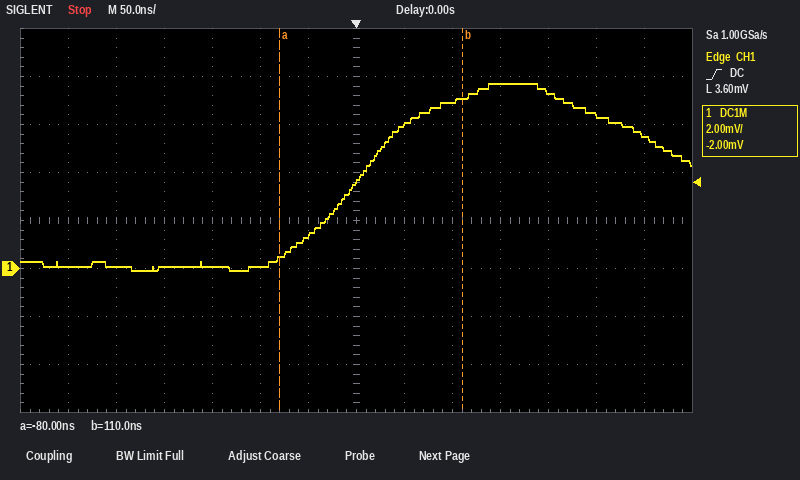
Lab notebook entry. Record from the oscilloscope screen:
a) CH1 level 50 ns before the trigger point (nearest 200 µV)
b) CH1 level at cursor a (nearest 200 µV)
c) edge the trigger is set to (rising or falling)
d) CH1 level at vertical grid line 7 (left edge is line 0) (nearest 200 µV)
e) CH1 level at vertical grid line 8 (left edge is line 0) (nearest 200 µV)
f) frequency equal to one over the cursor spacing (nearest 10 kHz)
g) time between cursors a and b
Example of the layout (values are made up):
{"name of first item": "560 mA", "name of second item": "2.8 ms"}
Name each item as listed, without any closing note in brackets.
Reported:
{"CH1 level 50 ns before the trigger point": "1.4 mV", "CH1 level at cursor a": "400 µV", "edge the trigger is set to": "rising", "CH1 level at vertical grid line 7 (left edge is line 0)": "3.6 mV", "CH1 level at vertical grid line 8 (left edge is line 0)": "6.0 mV", "frequency equal to one over the cursor spacing": "5.26 MHz", "time between cursors a and b": "190 ns"}
